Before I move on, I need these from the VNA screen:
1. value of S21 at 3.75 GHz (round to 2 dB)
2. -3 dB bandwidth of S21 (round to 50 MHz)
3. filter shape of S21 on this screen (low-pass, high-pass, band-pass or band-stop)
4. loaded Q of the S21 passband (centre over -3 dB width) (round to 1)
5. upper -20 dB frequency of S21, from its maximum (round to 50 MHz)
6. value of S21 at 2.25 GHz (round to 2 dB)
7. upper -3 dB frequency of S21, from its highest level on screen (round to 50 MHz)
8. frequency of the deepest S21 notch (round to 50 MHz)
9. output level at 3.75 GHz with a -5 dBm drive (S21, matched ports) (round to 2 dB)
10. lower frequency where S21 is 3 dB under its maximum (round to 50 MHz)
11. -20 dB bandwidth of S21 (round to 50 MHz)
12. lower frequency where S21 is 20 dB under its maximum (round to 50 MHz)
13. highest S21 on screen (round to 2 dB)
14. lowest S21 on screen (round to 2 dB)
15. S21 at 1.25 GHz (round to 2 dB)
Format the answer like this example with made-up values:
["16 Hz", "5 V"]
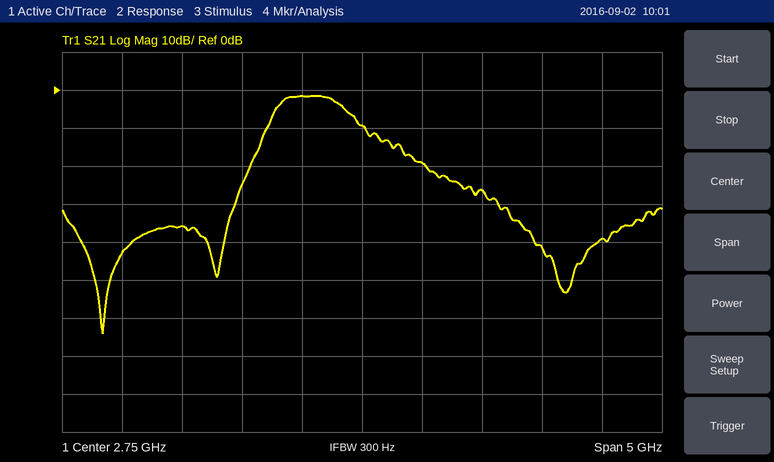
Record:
["-26 dB", "550 MHz", "band-pass", "4", "3.35 GHz", "-2 dB", "2.60 GHz", "600 MHz", "-32 dBm", "2.05 GHz", "1.55 GHz", "1.80 GHz", "-2 dB", "-64 dB", "-36 dB"]
